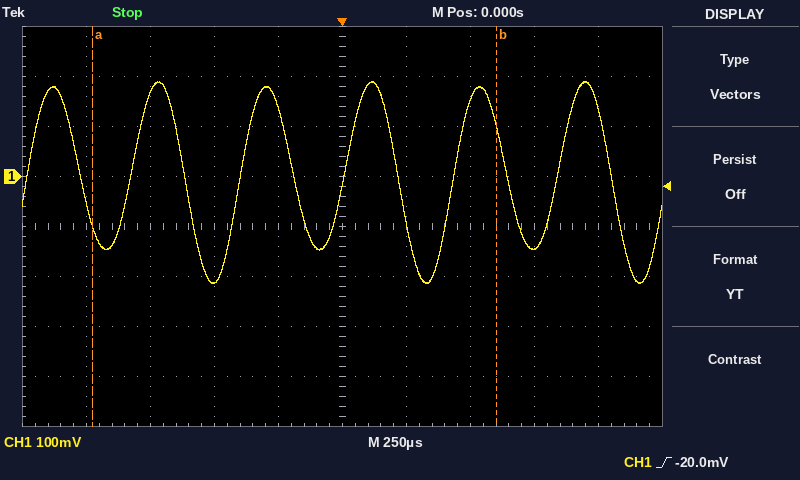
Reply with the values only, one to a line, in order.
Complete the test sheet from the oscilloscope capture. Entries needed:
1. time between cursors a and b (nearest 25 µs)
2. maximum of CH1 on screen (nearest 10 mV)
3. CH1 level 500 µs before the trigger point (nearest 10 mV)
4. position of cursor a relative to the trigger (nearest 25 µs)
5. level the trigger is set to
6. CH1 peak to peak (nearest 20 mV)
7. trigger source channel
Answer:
1.575 ms
190 mV
-210 mV
-975 µs
-20.0 mV
400 mV
CH1
